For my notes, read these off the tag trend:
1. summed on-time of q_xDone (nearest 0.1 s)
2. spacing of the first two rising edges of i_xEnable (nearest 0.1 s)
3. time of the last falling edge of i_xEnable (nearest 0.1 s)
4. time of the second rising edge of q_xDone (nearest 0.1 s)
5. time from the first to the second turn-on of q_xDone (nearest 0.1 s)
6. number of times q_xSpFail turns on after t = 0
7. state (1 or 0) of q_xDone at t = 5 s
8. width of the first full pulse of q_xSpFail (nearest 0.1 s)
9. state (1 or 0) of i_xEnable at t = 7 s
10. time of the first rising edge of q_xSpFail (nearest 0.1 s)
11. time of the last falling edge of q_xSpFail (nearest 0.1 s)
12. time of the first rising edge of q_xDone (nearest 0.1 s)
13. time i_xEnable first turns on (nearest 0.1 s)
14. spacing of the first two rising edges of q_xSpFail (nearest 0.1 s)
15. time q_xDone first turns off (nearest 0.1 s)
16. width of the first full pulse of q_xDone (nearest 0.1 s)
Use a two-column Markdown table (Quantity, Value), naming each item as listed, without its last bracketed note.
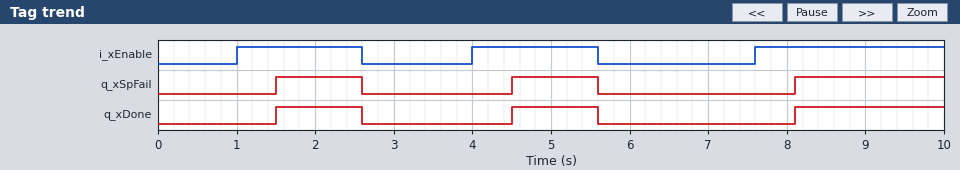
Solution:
| Quantity | Value |
|---|---|
| summed on-time of q_xDone | 4.1 s |
| spacing of the first two rising edges of i_xEnable | 3.0 s |
| time of the last falling edge of i_xEnable | 5.6 s |
| time of the second rising edge of q_xDone | 4.5 s |
| time from the first to the second turn-on of q_xDone | 3.0 s |
| number of times q_xSpFail turns on after t = 0 | 3 |
| state (1 or 0) of q_xDone at t = 5 s | 1 |
| width of the first full pulse of q_xSpFail | 1.1 s |
| state (1 or 0) of i_xEnable at t = 7 s | 0 |
| time of the first rising edge of q_xSpFail | 1.5 s |
| time of the last falling edge of q_xSpFail | 5.6 s |
| time of the first rising edge of q_xDone | 1.5 s |
| time i_xEnable first turns on | 1.0 s |
| spacing of the first two rising edges of q_xSpFail | 3.0 s |
| time q_xDone first turns off | 2.6 s |
| width of the first full pulse of q_xDone | 1.1 s |
